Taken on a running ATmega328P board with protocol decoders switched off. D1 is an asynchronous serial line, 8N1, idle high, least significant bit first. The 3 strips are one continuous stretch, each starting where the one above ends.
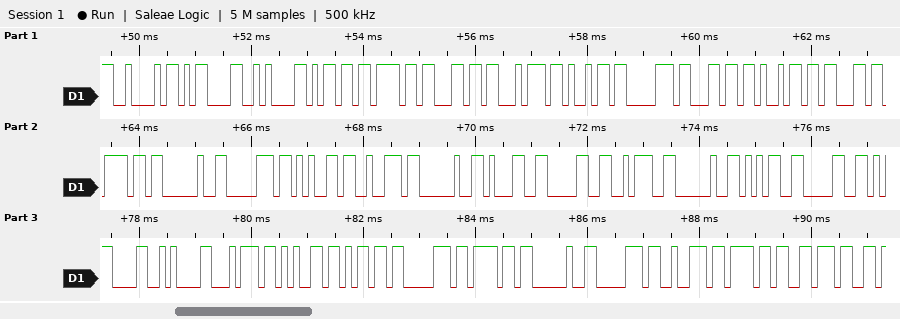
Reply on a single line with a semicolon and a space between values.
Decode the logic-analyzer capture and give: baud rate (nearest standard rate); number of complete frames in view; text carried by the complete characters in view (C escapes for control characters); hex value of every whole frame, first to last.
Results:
9600 baud; 36; "B\r\nmoltiplico per 10: 50\r\ntempo prov"; 42 0D 0A 6D 6F 6C 74 69 70 6C 69 63 6F 20 70 65 72 20 31 30 3A 20 35 30 0D 0A 74 65 6D 70 6F 20 70 72 6F 76
